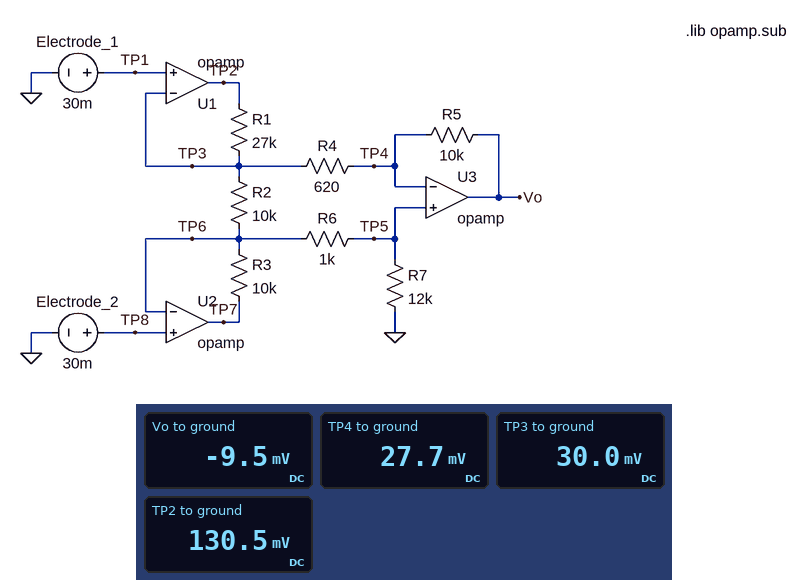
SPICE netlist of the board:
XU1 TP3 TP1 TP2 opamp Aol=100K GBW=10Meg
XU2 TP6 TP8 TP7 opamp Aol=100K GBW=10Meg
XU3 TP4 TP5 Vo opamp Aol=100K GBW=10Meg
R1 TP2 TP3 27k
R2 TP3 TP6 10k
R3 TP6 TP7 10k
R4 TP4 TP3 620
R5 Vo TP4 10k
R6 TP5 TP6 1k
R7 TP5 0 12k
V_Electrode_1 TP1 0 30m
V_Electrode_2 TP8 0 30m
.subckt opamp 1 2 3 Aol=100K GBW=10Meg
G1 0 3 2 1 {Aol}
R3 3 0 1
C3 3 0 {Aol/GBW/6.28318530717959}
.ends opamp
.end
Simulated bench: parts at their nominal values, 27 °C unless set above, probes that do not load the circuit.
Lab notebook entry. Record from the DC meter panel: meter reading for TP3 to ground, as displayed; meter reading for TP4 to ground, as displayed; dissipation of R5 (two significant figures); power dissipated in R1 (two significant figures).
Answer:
30.0 mV
27.7 mV
140 nW
370 nW
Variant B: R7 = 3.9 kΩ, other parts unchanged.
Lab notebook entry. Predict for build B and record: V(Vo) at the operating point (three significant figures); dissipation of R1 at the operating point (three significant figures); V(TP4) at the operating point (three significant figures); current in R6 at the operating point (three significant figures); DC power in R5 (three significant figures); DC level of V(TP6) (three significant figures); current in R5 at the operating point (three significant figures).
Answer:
-74.8 mV
2.63 µW
23.9 mV
6.12 µA
974 nW
30.0 mV
9.87 µA
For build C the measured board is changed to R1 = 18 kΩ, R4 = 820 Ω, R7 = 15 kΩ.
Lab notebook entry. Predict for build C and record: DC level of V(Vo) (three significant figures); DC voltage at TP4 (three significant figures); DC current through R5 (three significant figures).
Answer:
5.26 mV
28.1 mV
2.29 µA
